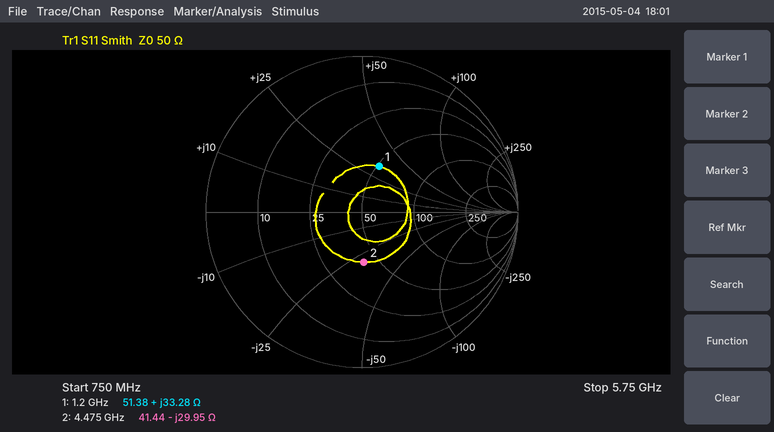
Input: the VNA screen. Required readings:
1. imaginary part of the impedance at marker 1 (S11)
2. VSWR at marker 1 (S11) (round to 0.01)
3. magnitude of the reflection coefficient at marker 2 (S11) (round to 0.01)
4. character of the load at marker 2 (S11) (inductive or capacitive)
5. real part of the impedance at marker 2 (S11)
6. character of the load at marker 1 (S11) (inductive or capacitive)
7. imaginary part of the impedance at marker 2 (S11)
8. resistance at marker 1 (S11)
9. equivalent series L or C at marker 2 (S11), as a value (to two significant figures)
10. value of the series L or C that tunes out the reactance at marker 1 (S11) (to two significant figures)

+33.28 Ω
1.91
0.32
capacitive
41.44 Ω
inductive
-29.95 Ω
51.38 Ω
1.2 pF
4.0 pF
